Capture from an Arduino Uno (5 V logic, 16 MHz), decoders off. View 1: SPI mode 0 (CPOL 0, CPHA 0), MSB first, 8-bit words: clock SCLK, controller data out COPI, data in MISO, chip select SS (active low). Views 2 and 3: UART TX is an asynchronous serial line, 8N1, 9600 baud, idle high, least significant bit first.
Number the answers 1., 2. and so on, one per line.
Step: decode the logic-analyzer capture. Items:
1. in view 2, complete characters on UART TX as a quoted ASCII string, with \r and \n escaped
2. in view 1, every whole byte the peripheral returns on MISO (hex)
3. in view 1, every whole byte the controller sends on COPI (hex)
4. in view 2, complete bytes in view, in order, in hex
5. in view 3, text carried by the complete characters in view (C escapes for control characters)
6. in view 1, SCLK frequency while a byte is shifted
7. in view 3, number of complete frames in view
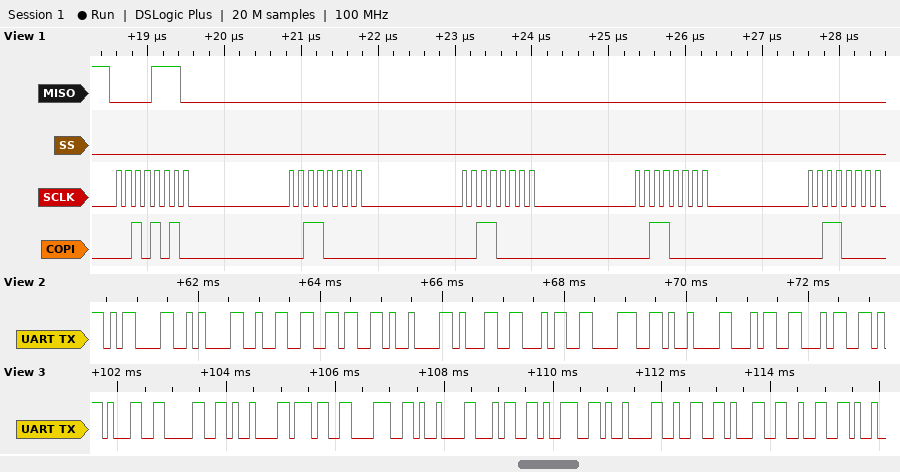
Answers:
1. "\r\n26\t148\t44"
2. 0E 00 00 00 00
3. 2A 30 30 30 30
4. 0D 0A 32 36 09 31 34 38 09 34 34
5. "10\t78\t49\t212"
6. 8 MHz
7. 12
